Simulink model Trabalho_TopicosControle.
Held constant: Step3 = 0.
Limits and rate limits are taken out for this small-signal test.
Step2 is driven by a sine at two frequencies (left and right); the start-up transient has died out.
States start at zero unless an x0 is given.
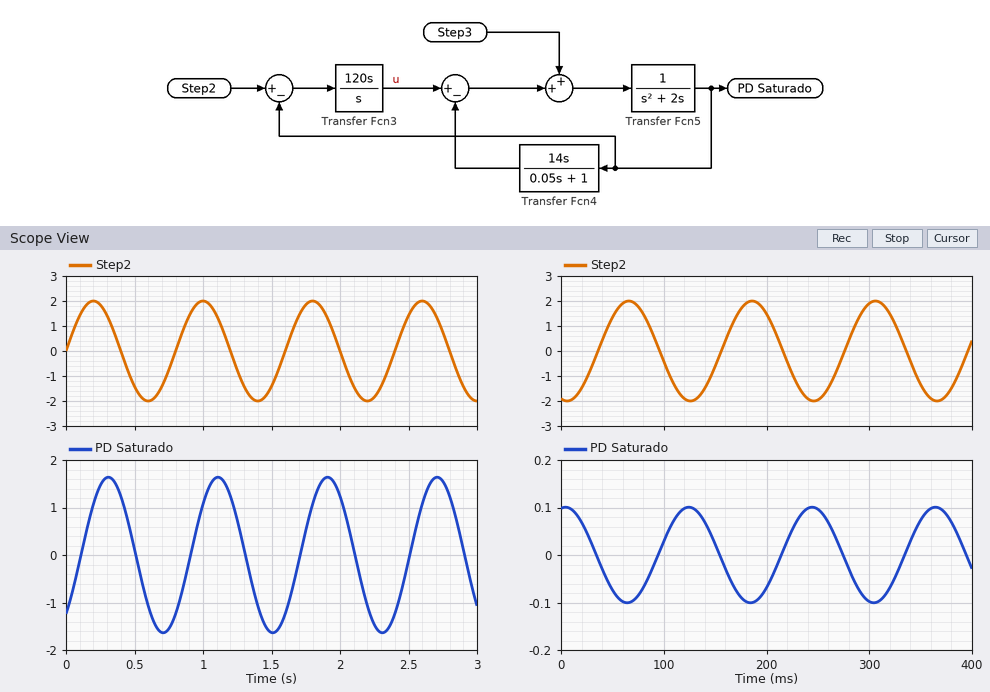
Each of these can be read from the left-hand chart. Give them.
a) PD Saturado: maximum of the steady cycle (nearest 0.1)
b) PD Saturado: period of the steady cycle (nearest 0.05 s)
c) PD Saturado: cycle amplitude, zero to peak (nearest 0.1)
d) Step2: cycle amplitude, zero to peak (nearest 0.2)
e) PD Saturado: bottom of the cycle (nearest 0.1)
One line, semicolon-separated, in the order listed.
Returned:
1.6; 0.80 s; 1.6; 2.0; -1.6
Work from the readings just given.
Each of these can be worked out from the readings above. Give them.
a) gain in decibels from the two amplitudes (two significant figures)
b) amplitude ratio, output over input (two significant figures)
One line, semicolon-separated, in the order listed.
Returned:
-1.9 dB; 0.80
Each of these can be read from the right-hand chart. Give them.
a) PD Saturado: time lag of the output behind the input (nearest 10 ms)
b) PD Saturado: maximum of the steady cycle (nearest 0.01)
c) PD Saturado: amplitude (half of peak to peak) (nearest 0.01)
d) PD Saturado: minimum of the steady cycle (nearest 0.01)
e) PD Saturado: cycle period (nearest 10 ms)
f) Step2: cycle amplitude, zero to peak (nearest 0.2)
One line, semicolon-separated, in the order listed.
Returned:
60 ms; 0.10; 0.10; -0.10; 120 ms; 2.0
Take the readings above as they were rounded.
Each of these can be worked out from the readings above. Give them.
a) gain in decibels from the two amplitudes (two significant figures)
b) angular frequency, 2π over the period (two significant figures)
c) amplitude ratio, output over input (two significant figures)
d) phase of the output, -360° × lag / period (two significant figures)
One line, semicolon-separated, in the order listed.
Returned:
-26 dB; 0.052 rad/ms; 0.050; -180°
